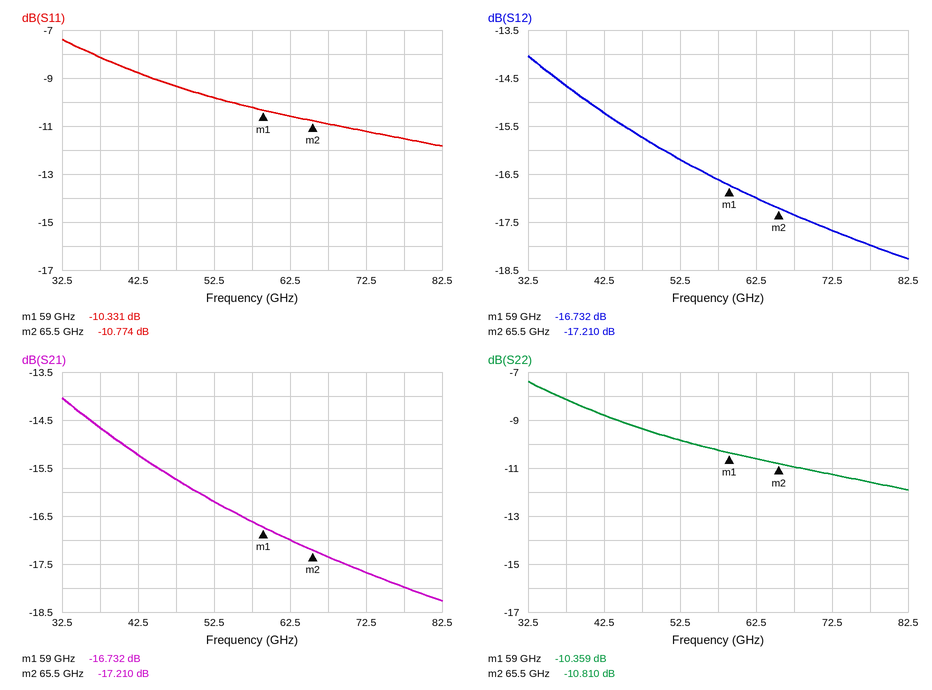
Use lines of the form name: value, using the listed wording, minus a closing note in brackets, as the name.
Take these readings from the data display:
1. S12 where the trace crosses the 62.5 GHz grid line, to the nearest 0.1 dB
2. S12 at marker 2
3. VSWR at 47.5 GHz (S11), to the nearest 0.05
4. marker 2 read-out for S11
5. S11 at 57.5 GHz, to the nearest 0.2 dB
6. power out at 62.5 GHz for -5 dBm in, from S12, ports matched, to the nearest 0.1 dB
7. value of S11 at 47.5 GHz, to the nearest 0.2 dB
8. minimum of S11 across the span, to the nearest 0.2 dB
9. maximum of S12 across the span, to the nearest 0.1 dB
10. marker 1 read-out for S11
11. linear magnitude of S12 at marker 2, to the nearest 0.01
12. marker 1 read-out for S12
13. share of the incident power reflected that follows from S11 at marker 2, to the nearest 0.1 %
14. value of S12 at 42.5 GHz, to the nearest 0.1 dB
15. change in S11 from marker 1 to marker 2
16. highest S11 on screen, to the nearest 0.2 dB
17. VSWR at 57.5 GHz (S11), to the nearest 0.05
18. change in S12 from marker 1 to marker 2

S12 where the trace crosses the 62.5 GHz grid line, to the nearest 0.1 dB: -17.0 dB
S12 at marker 2: -17.210 dB
VSWR at 47.5 GHz (S11), to the nearest 0.05: 2.05
marker 2 read-out for S11: -10.774 dB
S11 at 57.5 GHz, to the nearest 0.2 dB: -10.2 dB
power out at 62.5 GHz for -5 dBm in, from S12, ports matched, to the nearest 0.1 dB: -22.0 dBm
value of S11 at 47.5 GHz, to the nearest 0.2 dB: -9.4 dB
minimum of S11 across the span, to the nearest 0.2 dB: -11.8 dB
maximum of S12 across the span, to the nearest 0.1 dB: -14.0 dB
marker 1 read-out for S11: -10.331 dB
linear magnitude of S12 at marker 2, to the nearest 0.01: 0.14
marker 1 read-out for S12: -16.732 dB
share of the incident power reflected that follows from S11 at marker 2, to the nearest 0.1 %: 8.4 %
value of S12 at 42.5 GHz, to the nearest 0.1 dB: -15.2 dB
change in S11 from marker 1 to marker 2: -0.443 dB
highest S11 on screen, to the nearest 0.2 dB: -7.4 dB
VSWR at 57.5 GHz (S11), to the nearest 0.05: 1.90
change in S12 from marker 1 to marker 2: -0.478 dB
